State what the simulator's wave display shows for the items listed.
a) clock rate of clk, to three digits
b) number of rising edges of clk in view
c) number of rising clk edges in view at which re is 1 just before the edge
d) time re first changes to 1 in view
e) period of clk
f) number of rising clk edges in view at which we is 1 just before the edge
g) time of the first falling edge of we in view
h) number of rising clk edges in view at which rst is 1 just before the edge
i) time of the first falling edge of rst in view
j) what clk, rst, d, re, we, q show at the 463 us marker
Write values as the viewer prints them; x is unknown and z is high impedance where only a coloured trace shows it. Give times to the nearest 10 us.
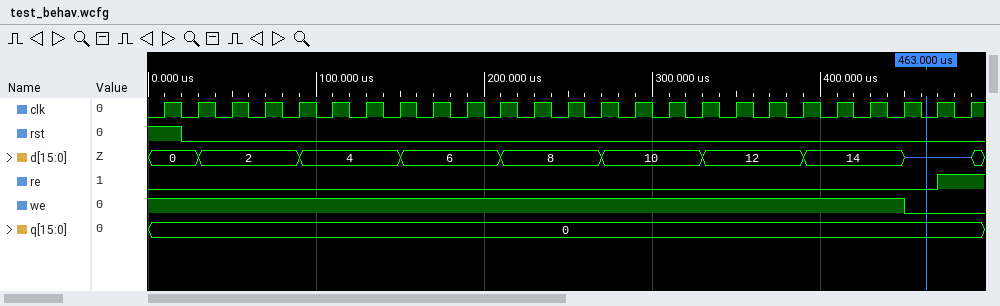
50.0 kHz
25
1
470 us
20 us
23
450 us
1
20 us
clk=0, rst=0, d=z, re=0, we=0, q=0
